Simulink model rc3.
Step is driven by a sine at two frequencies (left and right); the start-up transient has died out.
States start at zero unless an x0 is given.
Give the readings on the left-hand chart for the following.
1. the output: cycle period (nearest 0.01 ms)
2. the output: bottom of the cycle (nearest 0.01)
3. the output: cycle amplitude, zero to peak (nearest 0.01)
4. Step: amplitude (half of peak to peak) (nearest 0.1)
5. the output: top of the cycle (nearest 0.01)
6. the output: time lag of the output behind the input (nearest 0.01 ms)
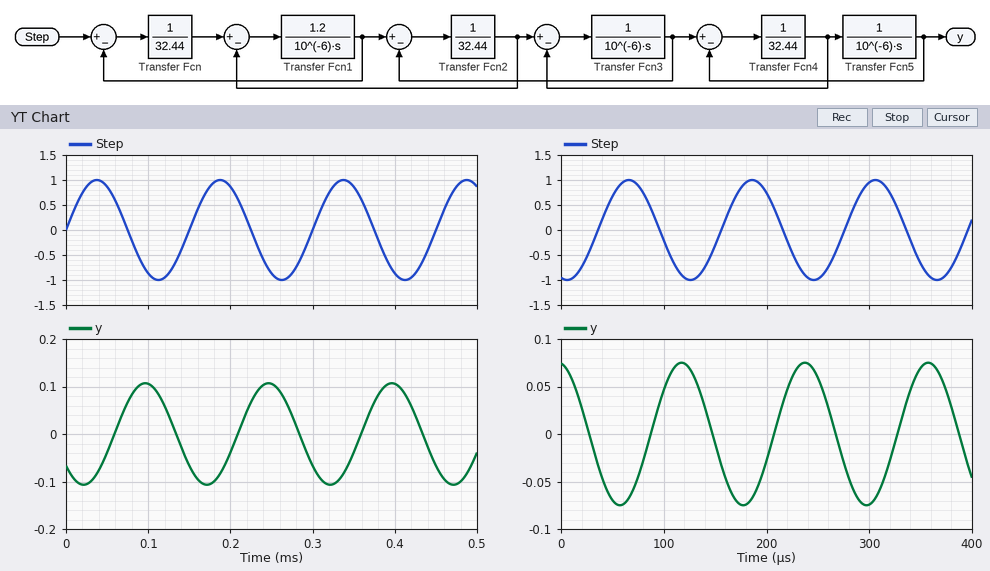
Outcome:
0.15 ms
-0.11
0.11
1.0
0.11
0.06 ms
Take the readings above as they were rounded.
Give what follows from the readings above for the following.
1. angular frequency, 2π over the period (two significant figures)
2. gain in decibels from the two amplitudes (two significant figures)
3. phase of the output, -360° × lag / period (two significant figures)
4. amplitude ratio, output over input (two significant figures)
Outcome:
42 rad/ms
-19 dB
-140°
0.11
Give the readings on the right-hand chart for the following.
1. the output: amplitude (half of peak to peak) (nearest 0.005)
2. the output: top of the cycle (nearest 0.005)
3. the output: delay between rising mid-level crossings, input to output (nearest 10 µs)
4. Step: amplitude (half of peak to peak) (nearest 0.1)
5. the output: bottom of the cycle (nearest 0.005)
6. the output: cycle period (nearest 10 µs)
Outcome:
0.075
0.075
50 µs
1.0
-0.075
120 µs
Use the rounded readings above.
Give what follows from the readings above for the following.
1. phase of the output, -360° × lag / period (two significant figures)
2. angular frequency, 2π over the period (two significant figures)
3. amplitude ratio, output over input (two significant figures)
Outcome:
-150°
0.052 rad/µs
0.075
